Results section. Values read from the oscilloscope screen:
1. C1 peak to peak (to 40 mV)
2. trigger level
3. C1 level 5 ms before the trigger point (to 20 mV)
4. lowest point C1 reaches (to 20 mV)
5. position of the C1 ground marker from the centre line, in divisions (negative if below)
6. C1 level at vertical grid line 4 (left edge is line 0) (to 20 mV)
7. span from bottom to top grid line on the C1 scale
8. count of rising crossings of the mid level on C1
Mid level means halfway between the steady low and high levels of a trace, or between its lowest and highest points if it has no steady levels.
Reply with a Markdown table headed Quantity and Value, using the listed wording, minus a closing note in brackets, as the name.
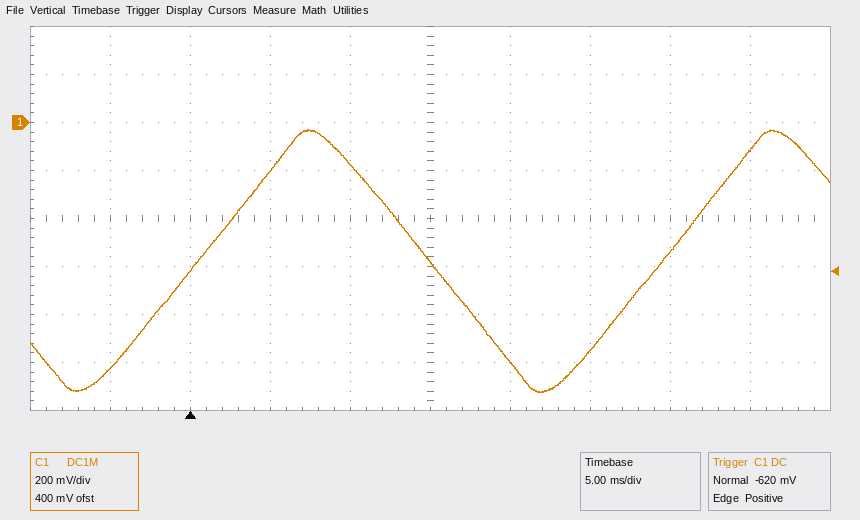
| Quantity | Value |
|---|---|
| C1 peak to peak | 1.08 V |
| trigger level | -620 mV |
| C1 level 5 ms before the trigger point | -1.02 V |
| lowest point C1 reaches | -1.12 V |
| position of the C1 ground marker from the centre line, in divisions | +2.0 div |
| C1 level at vertical grid line 4 (left edge is line 0) | -180 mV |
| span from bottom to top grid line on the C1 scale | 1.6 V |
| count of rising crossings of the mid level on C1 | 2 |
